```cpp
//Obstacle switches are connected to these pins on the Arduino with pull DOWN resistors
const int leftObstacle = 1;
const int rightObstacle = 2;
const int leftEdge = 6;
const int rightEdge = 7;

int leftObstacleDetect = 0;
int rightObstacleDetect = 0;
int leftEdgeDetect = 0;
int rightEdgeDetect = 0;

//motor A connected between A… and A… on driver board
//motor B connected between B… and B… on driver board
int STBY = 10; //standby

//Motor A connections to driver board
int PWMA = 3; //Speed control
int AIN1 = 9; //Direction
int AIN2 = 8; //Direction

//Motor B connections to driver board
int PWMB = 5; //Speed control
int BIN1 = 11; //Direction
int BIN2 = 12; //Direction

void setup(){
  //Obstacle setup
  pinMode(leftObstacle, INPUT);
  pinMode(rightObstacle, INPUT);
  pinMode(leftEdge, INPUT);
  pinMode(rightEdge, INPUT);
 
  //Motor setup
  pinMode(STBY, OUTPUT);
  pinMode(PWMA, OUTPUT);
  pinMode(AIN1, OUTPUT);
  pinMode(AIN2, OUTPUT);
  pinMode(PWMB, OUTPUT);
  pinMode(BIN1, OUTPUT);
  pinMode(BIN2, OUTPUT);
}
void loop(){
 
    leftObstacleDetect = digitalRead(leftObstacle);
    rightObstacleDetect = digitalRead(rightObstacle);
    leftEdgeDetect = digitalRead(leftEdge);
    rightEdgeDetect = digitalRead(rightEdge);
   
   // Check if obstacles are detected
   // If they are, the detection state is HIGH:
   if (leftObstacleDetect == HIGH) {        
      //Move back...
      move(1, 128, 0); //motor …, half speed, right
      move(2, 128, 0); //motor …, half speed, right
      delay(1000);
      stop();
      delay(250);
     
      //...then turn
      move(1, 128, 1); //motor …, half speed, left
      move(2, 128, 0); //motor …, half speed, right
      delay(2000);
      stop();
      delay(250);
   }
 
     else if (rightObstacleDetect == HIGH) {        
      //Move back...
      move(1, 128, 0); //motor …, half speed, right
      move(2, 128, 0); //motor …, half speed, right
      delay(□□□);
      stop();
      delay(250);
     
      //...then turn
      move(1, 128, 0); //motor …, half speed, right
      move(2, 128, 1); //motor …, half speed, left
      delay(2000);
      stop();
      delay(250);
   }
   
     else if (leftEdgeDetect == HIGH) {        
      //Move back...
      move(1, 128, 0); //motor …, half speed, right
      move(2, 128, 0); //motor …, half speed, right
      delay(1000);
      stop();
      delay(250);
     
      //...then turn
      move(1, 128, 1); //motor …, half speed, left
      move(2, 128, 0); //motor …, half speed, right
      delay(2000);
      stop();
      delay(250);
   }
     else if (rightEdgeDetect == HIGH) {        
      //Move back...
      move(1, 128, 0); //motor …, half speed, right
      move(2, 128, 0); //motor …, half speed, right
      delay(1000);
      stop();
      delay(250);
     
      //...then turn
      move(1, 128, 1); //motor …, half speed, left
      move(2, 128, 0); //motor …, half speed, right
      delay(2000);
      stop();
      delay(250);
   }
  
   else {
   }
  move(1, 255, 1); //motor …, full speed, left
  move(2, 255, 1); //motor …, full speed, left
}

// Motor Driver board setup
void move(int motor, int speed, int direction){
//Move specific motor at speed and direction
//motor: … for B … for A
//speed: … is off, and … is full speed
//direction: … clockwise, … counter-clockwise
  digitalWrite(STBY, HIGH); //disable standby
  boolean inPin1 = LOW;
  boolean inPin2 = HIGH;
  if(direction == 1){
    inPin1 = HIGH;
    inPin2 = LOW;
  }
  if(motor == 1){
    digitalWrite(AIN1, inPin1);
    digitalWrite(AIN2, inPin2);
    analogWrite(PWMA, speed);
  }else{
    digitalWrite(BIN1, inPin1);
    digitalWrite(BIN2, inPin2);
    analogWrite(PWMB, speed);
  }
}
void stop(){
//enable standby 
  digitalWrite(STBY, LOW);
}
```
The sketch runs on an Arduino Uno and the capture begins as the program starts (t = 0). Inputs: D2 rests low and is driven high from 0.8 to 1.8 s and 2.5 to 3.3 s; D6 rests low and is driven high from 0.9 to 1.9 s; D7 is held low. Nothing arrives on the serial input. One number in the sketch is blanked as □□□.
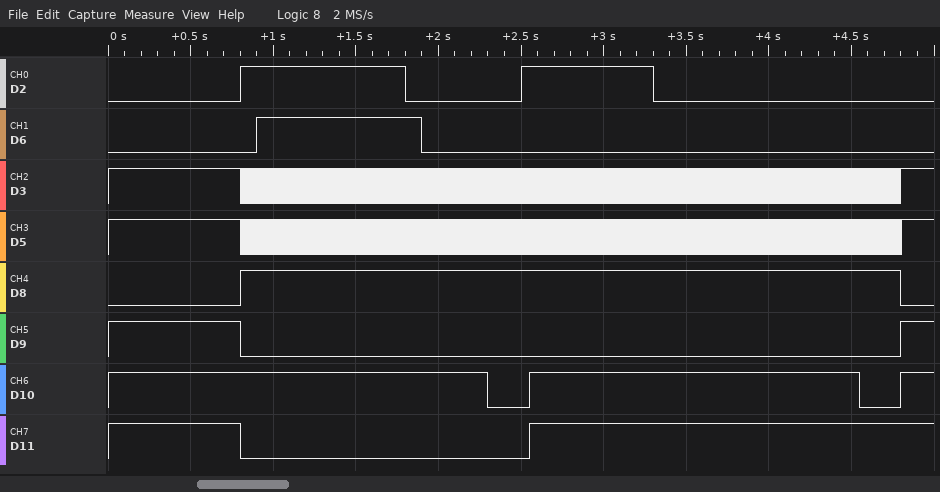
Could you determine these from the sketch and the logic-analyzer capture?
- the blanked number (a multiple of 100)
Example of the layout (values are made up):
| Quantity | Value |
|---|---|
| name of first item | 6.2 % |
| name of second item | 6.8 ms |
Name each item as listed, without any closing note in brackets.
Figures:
| Quantity | Value |
|---|---|
| the blanked number | 1500 |
